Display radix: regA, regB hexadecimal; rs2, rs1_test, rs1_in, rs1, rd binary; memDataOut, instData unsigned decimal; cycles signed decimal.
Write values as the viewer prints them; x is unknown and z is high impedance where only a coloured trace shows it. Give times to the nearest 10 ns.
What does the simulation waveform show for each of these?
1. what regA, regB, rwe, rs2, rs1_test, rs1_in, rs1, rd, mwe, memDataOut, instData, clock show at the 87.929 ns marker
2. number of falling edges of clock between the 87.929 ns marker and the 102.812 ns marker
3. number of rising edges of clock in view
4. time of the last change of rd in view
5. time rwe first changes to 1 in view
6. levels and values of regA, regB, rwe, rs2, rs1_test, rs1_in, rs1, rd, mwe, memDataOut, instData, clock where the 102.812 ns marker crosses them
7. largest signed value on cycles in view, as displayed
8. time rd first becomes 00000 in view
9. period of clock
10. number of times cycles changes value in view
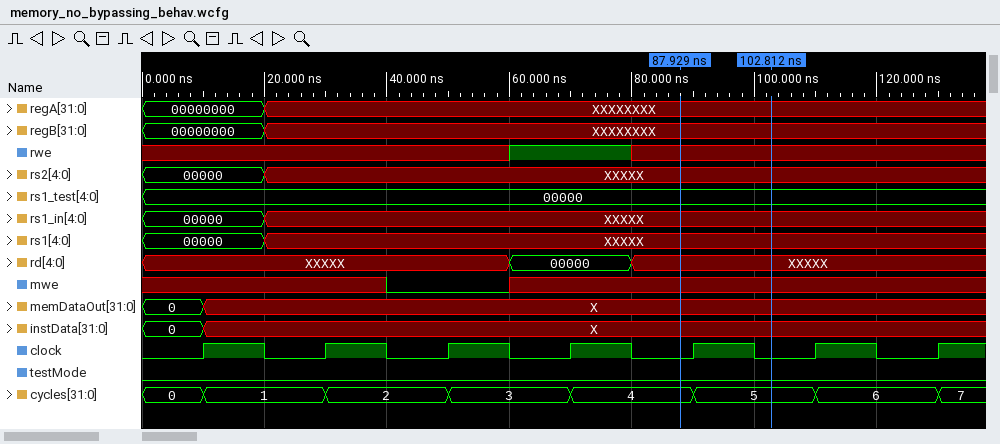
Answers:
regA=XXXXXXXX, regB=XXXXXXXX, rwe=x, rs2=XXXXX, rs1_test=00000, rs1_in=XXXXX, rs1=XXXXX, rd=XXXXX, mwe=x, memDataOut=X, instData=X, clock=0
1
7
80 ns
60 ns
regA=XXXXXXXX, regB=XXXXXXXX, rwe=x, rs2=XXXXX, rs1_test=00000, rs1_in=XXXXX, rs1=XXXXX, rd=XXXXX, mwe=x, memDataOut=X, instData=X, clock=0
7
60 ns
20 ns
7
